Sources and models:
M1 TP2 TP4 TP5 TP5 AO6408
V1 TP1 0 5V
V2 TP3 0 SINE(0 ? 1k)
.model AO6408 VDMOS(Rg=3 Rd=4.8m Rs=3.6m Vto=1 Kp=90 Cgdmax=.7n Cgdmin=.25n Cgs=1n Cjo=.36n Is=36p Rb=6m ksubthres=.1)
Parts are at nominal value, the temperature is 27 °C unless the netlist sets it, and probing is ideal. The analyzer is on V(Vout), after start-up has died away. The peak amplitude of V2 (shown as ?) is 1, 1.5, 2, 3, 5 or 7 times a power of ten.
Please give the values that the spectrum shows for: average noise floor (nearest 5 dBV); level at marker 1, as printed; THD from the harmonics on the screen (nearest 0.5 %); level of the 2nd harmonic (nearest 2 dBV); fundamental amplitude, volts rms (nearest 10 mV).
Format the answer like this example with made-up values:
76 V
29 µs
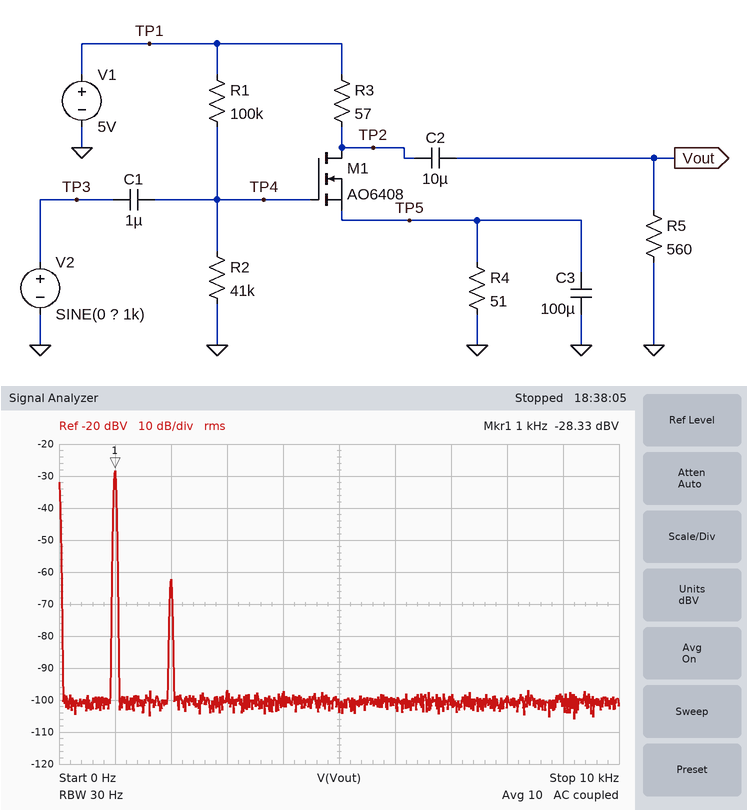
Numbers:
-100 dBV
-28.33 dBV
2.0 %
-62 dBV
40 mV
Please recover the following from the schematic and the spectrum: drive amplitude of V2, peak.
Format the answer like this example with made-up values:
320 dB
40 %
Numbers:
5 mV
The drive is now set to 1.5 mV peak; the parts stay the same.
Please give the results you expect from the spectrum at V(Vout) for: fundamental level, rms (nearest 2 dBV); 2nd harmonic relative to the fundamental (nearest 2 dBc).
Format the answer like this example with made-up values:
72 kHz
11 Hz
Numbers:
-38 dBV
-44 dBc
